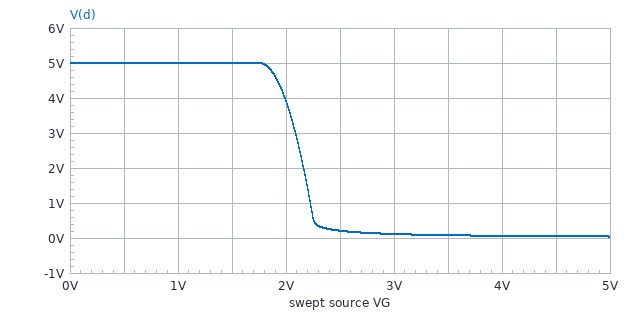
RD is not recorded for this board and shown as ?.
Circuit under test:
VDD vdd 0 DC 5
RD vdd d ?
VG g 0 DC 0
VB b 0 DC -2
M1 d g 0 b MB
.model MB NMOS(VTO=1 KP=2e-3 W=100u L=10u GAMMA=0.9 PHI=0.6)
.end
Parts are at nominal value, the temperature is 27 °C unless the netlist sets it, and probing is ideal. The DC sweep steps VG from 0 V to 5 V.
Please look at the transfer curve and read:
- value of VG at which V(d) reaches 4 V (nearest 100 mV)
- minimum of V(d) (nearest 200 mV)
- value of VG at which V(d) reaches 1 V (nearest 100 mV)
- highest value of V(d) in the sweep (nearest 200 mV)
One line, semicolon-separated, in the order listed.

2.0 V; 0 V; 2.2 V; 5.0 V
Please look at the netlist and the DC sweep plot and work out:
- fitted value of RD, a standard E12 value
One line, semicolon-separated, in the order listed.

1.8 kΩ
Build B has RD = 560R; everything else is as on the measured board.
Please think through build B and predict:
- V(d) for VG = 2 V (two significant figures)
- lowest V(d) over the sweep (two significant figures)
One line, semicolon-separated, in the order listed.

4.7 V; 140 mV
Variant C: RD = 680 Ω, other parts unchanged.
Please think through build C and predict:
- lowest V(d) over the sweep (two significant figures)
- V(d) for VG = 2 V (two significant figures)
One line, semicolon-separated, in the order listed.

110 mV; 4.6 V
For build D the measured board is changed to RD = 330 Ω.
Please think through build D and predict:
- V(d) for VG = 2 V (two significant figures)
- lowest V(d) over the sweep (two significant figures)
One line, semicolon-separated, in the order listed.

4.8 V; 230 mV
